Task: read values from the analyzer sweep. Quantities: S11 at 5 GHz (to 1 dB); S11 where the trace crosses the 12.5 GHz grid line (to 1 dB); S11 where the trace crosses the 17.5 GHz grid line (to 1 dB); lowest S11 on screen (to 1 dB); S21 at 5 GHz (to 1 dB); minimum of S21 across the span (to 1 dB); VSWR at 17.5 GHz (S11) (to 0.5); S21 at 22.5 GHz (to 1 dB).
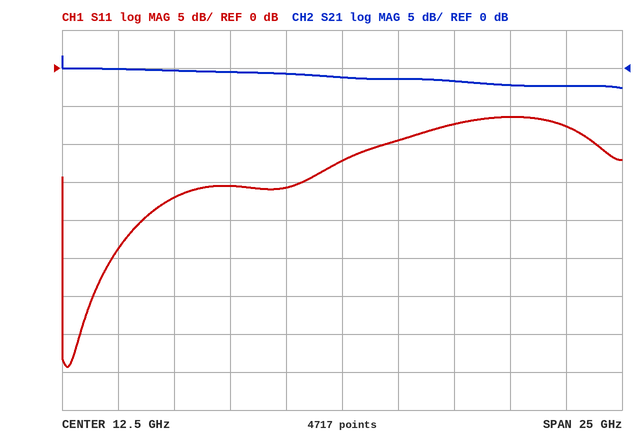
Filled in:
-17 dB
-12 dB
-7 dB
-39 dB
0 dB
-3 dB
2.5
-2 dB
